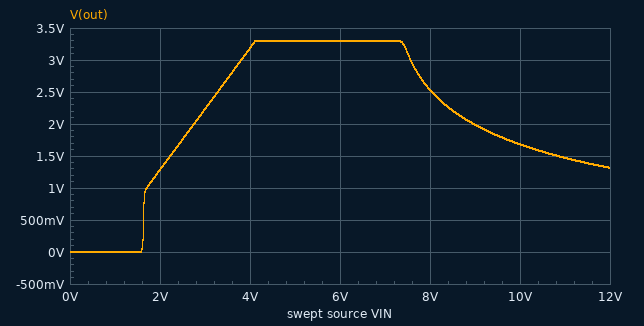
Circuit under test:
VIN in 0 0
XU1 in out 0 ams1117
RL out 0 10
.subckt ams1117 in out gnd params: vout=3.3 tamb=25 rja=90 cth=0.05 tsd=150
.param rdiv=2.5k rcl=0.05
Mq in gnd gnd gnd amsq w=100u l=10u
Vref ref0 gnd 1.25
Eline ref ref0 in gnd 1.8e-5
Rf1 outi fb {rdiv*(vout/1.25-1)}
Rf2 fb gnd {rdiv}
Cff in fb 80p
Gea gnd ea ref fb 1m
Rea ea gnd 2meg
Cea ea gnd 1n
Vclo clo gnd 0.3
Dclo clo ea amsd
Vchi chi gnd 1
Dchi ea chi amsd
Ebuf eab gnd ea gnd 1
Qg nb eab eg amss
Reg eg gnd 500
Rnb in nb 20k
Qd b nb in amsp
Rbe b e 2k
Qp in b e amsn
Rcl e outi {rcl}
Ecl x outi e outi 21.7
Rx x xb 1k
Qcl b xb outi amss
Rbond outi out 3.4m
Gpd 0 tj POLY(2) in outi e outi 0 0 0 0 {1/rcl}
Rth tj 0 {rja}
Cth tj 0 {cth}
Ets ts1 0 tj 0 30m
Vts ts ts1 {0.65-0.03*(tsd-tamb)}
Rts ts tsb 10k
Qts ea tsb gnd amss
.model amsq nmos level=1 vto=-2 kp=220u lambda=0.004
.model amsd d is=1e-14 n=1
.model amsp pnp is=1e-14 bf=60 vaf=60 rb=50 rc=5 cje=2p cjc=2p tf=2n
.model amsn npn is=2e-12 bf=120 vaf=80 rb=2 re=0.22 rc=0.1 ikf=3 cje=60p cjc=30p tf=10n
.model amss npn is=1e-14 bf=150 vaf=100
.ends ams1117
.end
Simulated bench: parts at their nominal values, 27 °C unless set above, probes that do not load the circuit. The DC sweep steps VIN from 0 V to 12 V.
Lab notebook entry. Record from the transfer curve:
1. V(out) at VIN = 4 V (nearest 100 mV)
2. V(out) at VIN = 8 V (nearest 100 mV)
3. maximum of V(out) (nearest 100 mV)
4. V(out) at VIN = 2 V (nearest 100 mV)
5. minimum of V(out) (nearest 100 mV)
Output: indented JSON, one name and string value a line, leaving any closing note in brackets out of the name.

{
  "V(out) at VIN = 4 V": "3.2 V",
  "V(out) at VIN = 8 V": "2.5 V",
  "maximum of V(out)": "3.3 V",
  "V(out) at VIN = 2 V": "1.3 V",
  "minimum of V(out)": "0 V"
}
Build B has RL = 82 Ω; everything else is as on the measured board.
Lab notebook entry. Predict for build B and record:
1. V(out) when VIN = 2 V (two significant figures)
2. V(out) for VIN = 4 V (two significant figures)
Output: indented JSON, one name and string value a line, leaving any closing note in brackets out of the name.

{
  "V(out) when VIN = 2 V": "1.4 V",
  "V(out) for VIN = 4 V": "3.3 V"
}
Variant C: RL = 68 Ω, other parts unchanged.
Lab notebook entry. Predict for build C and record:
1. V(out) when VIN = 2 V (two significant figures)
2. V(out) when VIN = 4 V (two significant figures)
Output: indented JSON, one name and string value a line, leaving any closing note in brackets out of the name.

{
  "V(out) when VIN = 2 V": "1.4 V",
  "V(out) when VIN = 4 V": "3.3 V"
}
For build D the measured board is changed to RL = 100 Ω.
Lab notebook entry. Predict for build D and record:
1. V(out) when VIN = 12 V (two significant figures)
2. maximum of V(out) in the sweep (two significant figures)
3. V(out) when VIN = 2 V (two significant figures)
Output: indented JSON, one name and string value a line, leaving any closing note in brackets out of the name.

{
  "V(out) when VIN = 12 V": "3.3 V",
  "maximum of V(out) in the sweep": "3.3 V",
  "V(out) when VIN = 2 V": "1.4 V"
}
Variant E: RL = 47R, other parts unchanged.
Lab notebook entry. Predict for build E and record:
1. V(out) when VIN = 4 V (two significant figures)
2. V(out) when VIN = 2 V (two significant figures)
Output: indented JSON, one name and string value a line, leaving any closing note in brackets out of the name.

{
  "V(out) when VIN = 4 V": "3.3 V",
  "V(out) when VIN = 2 V": "1.4 V"
}
